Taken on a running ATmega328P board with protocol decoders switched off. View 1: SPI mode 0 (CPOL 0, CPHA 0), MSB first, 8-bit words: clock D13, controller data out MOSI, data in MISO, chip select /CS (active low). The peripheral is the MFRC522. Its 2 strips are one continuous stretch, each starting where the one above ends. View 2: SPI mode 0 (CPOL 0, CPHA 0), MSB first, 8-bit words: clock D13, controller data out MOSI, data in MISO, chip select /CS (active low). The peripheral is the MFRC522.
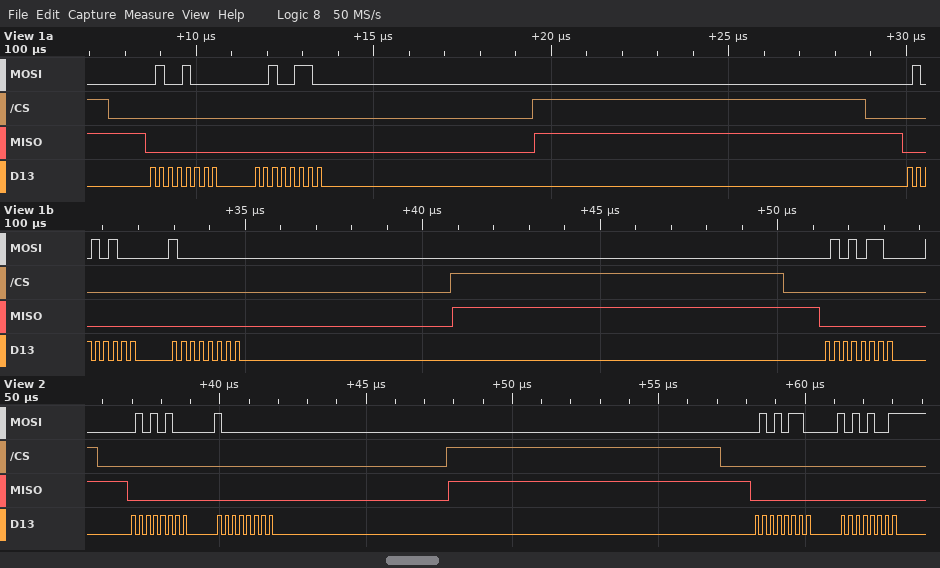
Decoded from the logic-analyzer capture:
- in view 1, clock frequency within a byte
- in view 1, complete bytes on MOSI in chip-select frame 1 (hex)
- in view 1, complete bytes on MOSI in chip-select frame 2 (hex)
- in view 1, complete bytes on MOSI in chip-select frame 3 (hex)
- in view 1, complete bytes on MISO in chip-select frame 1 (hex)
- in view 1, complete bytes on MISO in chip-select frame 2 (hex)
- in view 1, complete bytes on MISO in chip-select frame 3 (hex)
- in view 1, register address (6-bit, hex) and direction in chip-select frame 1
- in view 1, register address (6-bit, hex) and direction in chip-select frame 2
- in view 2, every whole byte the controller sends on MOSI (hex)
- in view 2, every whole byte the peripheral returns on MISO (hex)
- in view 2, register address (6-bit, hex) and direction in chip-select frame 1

4 MHz
48 26
54 80
56
00 00
00 00
00
0x24 write
0x2A write
54 80 56 A9
00 00 00 00
0x2A write
